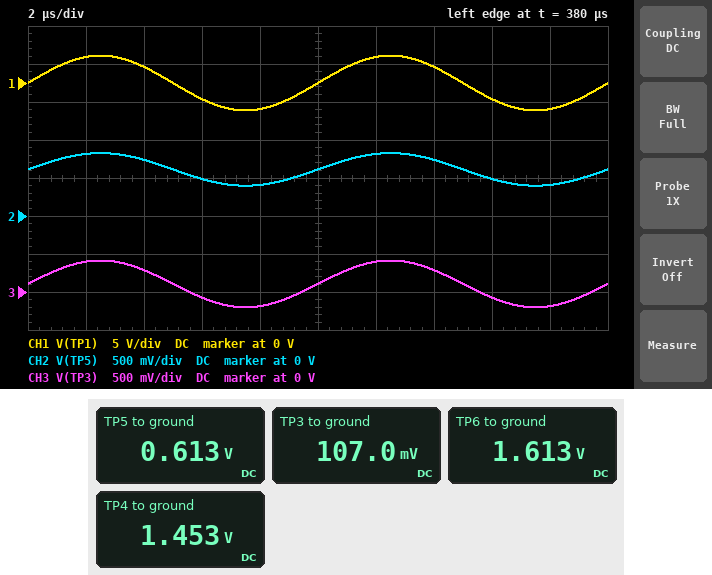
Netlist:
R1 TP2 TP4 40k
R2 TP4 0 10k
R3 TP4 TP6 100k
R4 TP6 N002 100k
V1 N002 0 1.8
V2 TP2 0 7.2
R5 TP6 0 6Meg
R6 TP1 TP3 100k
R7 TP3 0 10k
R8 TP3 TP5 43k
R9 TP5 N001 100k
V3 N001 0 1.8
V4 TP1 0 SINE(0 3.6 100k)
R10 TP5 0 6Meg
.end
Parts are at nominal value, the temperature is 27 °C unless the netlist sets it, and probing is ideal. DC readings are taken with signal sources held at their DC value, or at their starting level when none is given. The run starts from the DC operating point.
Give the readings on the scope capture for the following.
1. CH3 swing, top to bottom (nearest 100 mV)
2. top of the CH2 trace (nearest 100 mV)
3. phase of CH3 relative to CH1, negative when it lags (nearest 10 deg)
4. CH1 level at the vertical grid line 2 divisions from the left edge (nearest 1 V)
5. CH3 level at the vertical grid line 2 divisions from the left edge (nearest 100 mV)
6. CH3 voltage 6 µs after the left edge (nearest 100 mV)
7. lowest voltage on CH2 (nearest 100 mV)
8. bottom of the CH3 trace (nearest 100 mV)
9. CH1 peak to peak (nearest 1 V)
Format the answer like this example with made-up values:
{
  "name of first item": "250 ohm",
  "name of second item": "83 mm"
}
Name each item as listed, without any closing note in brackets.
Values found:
{
  "CH3 swing, top to bottom": "600 mV",
  "top of the CH2 trace": "800 mV",
  "phase of CH3 relative to CH1, negative when it lags": "0 deg",
  "CH1 level at the vertical grid line 2 divisions from the left edge": "2 V",
  "CH3 level at the vertical grid line 2 divisions from the left edge": "300 mV",
  "CH3 voltage 6 µs after the left edge": "-100 mV",
  "lowest voltage on CH2": "400 mV",
  "bottom of the CH3 trace": "-200 mV",
  "CH1 peak to peak": "7 V"
}
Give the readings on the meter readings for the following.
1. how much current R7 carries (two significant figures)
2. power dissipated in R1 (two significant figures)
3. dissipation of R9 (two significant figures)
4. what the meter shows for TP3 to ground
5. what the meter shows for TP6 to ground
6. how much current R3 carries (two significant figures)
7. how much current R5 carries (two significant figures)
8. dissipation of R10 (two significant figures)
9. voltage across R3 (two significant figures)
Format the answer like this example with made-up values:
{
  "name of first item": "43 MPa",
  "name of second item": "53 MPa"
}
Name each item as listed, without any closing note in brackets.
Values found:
{
  "how much current R7 carries": "11 µA",
  "power dissipated in R1": "830 µW",
  "dissipation of R9": "14 µW",
  "what the meter shows for TP3 to ground": "107.0 mV",
  "what the meter shows for TP6 to ground": "1.613 V",
  "how much current R3 carries": "1.6 µA",
  "how much current R5 carries": "270 nA",
  "dissipation of R10": "63 nW",
  "voltage across R3": "160 mV"
}
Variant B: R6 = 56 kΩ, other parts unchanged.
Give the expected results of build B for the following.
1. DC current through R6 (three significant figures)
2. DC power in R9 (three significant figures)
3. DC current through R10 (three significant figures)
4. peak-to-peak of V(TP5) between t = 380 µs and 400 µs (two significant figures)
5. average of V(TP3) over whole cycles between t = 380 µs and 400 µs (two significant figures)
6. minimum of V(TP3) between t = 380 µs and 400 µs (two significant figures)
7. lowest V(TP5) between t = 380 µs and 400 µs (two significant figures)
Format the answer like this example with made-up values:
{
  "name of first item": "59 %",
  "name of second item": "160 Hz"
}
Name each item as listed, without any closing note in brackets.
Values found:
{
  "DC current through R6": "1.79 µA",
  "DC power in R9": "14.2 µW",
  "DC current through R10": "101 nA",
  "peak-to-peak of V(TP5) between t = 380 µs and 400 µs": "720 mV",
  "average of V(TP3) over whole cycles between t = 380 µs and 400 µs": "100 mV",
  "minimum of V(TP3) between t = 380 µs and 400 µs": "-410 mV",
  "lowest V(TP5) between t = 380 µs and 400 µs": "250 mV"
}
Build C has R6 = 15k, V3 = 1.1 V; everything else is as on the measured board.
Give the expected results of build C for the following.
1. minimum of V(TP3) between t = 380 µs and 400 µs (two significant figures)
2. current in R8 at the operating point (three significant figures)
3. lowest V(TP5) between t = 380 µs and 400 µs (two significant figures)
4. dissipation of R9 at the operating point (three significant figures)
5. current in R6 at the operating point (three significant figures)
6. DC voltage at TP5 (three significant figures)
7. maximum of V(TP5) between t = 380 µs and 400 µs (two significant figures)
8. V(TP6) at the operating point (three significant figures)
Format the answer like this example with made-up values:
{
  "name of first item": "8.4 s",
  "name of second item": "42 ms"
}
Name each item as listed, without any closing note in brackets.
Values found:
{
  "minimum of V(TP3) between t = 380 µs and 400 µs": "-1.3 V",
  "current in R8 at the operating point": "7.34 µA",
  "lowest V(TP5) between t = 380 µs and 400 µs": "-600 mV",
  "dissipation of R9 at the operating point": "5.48 µW",
  "current in R6 at the operating point": "2.94 µA",
  "DC voltage at TP5": "360 mV",
  "maximum of V(TP5) between t = 380 µs and 400 µs": "1.3 V",
  "V(TP6) at the operating point": "1.61 V"
}
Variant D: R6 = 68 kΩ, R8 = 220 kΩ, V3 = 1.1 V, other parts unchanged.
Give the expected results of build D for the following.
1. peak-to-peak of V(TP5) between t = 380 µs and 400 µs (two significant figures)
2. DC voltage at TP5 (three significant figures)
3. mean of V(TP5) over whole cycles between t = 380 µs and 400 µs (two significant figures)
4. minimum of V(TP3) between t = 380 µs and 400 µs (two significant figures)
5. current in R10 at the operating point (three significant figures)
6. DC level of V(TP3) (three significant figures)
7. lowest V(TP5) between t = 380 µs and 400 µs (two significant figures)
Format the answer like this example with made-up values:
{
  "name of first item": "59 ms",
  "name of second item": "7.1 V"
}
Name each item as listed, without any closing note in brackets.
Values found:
{
  "peak-to-peak of V(TP5) between t = 380 µs and 400 µs": "280 mV",
  "DC voltage at TP5": "757 mV",
  "mean of V(TP5) over whole cycles between t = 380 µs and 400 µs": "760 mV",
  "minimum of V(TP3) between t = 380 µs and 400 µs": "-420 mV",
  "current in R10 at the operating point": "126 nA",
  "DC level of V(TP3)": "28.8 mV",
  "lowest V(TP5) between t = 380 µs and 400 µs": "620 mV"
}
